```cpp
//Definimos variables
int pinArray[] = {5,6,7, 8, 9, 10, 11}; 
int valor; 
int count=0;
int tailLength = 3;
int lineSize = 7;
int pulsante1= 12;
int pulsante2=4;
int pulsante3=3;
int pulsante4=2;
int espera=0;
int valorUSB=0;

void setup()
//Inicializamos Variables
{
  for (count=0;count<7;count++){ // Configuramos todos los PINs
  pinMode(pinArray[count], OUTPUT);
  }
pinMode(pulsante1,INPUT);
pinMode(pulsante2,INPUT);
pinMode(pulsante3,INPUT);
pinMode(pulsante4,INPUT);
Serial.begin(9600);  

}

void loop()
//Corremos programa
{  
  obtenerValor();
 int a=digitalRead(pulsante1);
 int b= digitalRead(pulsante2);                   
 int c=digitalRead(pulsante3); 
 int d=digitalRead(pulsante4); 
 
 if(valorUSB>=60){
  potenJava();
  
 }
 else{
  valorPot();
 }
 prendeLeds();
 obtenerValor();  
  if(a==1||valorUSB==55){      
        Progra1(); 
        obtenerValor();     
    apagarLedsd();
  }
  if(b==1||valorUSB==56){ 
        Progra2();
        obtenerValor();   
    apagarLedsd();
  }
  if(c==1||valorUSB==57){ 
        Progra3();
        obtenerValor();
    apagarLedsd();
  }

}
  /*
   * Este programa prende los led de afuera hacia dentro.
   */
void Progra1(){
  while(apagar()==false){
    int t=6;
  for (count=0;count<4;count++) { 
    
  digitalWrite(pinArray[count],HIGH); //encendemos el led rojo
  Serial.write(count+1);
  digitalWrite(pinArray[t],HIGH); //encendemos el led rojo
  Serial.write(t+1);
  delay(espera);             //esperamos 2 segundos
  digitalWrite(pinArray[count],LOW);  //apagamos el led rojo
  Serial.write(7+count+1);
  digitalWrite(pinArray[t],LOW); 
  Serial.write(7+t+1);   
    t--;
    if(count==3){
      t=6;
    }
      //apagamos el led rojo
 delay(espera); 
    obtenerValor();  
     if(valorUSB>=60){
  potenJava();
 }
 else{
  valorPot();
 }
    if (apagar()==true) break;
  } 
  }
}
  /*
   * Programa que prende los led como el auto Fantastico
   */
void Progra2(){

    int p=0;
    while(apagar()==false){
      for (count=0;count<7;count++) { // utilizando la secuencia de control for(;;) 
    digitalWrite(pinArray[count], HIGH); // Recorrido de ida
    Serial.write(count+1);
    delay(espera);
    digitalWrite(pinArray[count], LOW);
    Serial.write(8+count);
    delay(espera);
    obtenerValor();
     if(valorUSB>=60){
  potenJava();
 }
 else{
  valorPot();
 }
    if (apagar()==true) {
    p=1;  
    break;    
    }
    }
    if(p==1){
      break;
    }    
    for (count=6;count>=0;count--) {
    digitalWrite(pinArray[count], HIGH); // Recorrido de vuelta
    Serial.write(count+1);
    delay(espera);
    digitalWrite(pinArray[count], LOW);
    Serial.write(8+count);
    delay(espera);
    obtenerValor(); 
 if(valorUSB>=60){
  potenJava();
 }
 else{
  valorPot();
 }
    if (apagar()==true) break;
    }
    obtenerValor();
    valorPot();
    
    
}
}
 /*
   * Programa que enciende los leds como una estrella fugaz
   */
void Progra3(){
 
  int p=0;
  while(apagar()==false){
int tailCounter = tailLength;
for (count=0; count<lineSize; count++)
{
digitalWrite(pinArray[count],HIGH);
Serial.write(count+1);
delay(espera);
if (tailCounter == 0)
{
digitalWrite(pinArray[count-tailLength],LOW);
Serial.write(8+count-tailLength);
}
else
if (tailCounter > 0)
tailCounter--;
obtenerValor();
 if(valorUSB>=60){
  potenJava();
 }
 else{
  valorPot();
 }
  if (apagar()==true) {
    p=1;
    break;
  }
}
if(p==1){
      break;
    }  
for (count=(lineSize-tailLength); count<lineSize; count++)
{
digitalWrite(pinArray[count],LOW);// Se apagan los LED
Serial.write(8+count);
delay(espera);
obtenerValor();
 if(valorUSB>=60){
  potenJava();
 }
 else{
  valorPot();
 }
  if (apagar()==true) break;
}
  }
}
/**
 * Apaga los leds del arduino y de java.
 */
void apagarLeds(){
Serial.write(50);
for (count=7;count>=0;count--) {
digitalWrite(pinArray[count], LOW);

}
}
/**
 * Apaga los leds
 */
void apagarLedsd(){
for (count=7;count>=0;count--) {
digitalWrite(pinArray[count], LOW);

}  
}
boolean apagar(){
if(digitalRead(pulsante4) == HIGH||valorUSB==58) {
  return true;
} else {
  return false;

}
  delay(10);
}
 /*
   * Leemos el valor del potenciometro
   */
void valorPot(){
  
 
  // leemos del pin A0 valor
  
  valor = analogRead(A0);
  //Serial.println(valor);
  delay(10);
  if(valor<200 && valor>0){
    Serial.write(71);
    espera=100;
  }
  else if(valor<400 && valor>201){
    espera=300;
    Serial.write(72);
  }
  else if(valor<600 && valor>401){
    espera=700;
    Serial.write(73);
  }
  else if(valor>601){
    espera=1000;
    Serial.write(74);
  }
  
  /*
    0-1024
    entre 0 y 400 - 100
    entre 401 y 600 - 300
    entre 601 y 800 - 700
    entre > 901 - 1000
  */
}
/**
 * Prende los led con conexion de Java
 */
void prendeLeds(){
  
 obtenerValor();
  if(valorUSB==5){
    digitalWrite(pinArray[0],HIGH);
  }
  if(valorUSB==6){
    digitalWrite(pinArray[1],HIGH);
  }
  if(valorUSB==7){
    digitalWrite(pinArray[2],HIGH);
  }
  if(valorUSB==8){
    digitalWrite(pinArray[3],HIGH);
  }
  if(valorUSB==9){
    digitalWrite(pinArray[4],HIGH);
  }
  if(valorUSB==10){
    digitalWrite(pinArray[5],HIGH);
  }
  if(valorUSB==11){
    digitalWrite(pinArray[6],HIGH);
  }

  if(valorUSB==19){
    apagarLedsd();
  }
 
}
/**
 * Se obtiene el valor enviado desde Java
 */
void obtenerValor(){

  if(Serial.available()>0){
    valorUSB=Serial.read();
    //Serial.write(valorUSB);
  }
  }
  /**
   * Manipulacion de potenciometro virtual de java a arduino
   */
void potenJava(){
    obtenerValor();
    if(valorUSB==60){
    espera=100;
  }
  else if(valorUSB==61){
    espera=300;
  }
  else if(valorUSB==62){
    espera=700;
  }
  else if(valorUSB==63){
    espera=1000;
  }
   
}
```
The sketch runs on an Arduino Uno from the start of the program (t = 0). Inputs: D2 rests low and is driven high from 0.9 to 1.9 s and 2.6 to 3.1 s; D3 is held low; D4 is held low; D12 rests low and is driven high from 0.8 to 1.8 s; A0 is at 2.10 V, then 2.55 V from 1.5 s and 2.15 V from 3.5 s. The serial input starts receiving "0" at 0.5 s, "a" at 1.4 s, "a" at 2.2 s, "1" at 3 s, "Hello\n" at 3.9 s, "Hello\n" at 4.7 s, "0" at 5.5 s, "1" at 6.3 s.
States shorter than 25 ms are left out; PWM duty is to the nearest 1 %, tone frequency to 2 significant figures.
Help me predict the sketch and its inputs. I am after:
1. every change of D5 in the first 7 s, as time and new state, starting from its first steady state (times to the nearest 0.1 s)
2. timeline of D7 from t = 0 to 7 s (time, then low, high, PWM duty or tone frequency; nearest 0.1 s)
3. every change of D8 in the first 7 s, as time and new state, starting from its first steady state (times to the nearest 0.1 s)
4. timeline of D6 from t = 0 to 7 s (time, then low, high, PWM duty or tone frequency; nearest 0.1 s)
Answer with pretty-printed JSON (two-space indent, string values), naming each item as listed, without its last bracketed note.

{
  "every change of D5 in the first 7 s, as time and new state, starting from its first steady state": "0 s low; 0.8 s high; 1.5 s low; 6.4 s high",
  "timeline of D7 from t = 0 to 7 s": "0 s low; 3.6 s high; 4.3 s low",
  "every change of D8 in the first 7 s, as time and new state, starting from its first steady state": "0 s low; 5 s high; 5.7 s low",
  "timeline of D6 from t = 0 to 7 s": "0 s low; 2.2 s high; 2.9 s low"
}
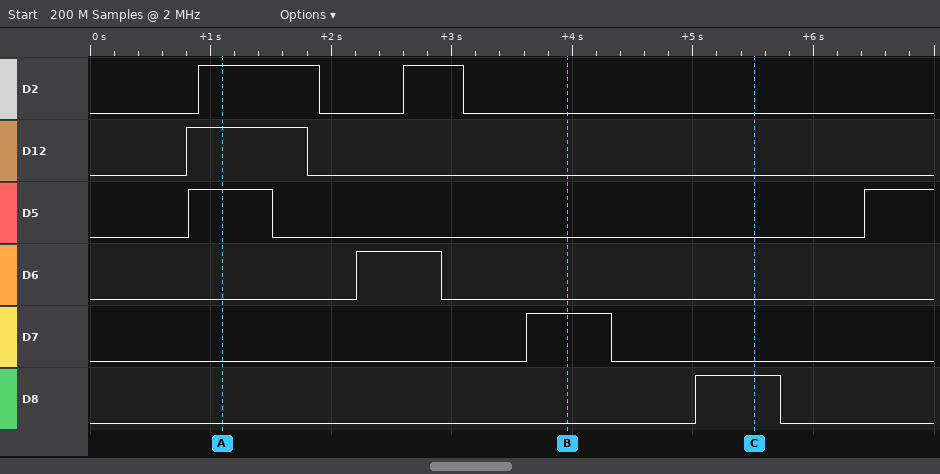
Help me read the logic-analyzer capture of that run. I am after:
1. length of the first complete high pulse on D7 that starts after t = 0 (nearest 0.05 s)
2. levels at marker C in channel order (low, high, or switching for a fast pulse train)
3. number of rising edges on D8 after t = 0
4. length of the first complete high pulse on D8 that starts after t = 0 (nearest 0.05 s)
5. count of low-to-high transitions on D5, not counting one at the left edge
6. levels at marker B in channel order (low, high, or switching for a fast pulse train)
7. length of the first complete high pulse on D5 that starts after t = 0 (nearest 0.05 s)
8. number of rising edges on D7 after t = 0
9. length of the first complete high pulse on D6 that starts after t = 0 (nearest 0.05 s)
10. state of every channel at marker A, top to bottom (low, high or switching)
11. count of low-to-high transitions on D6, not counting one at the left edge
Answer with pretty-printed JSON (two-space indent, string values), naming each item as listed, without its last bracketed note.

{
  "length of the first complete high pulse on D7 that starts after t = 0": "0.70 s",
  "levels at marker C in channel order": "D2 low, D12 low, D5 low, D6 low, D7 low, D8 high",
  "number of rising edges on D8 after t = 0": "1",
  "length of the first complete high pulse on D8 that starts after t = 0": "0.70 s",
  "count of low-to-high transitions on D5, not counting one at the left edge": "2",
  "levels at marker B in channel order": "D2 low, D12 low, D5 low, D6 low, D7 high, D8 low",
  "length of the first complete high pulse on D5 that starts after t = 0": "0.70 s",
  "number of rising edges on D7 after t = 0": "1",
  "length of the first complete high pulse on D6 that starts after t = 0": "0.70 s",
  "state of every channel at marker A, top to bottom": "D2 high, D12 high, D5 high, D6 low, D7 low, D8 low",
  "count of low-to-high transitions on D6, not counting one at the left edge": "1"
}
